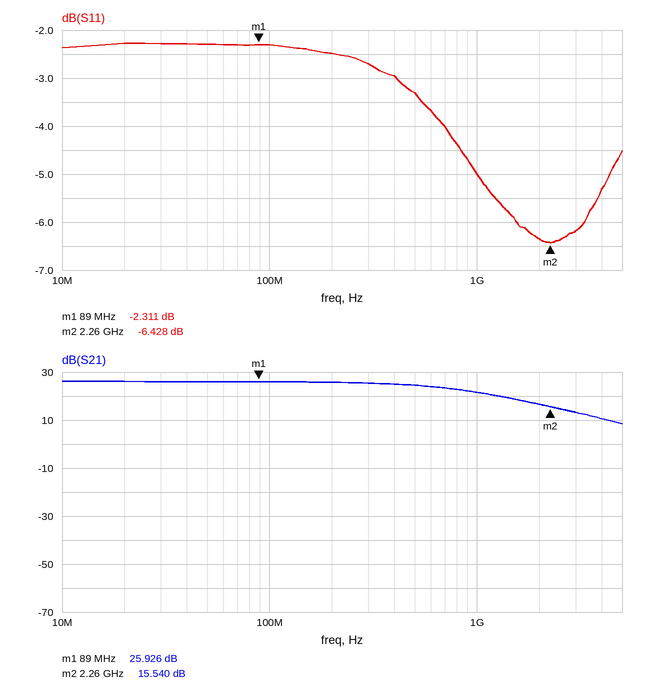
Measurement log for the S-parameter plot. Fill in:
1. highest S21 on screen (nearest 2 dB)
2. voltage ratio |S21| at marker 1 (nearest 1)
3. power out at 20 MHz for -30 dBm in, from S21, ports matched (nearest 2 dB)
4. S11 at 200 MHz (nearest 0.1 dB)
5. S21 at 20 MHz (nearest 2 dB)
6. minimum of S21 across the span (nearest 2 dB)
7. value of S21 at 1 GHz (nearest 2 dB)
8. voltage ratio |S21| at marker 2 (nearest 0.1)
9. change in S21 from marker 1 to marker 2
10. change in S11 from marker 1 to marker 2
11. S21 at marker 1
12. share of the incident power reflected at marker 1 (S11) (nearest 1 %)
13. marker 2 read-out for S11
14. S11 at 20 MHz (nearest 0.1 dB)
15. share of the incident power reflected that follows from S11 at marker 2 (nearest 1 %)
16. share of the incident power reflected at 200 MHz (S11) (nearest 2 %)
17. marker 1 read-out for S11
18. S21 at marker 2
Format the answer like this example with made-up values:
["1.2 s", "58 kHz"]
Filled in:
["26 dB", "20", "-4 dBm", "-2.5 dB", "26 dB", "8 dB", "22 dB", "6.0", "-10.386 dB", "-4.117 dB", "25.926 dB", "59 %", "-6.428 dB", "-2.3 dB", "23 %", "56 %", "-2.311 dB", "15.540 dB"]
